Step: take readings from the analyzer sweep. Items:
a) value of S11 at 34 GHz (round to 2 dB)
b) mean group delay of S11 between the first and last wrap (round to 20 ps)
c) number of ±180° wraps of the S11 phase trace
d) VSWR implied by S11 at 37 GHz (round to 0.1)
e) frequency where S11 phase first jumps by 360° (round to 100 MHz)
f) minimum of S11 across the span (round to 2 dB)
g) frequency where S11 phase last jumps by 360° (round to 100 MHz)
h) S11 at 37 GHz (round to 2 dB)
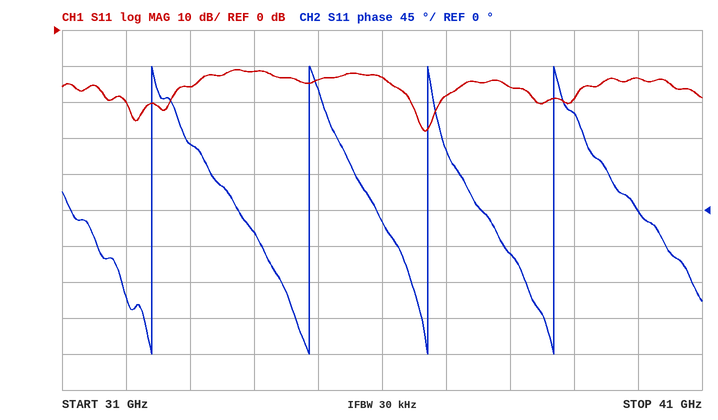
-12 dB
480 ps
4
1.3
32.4 GHz
-28 dB
38.7 GHz
-18 dB
